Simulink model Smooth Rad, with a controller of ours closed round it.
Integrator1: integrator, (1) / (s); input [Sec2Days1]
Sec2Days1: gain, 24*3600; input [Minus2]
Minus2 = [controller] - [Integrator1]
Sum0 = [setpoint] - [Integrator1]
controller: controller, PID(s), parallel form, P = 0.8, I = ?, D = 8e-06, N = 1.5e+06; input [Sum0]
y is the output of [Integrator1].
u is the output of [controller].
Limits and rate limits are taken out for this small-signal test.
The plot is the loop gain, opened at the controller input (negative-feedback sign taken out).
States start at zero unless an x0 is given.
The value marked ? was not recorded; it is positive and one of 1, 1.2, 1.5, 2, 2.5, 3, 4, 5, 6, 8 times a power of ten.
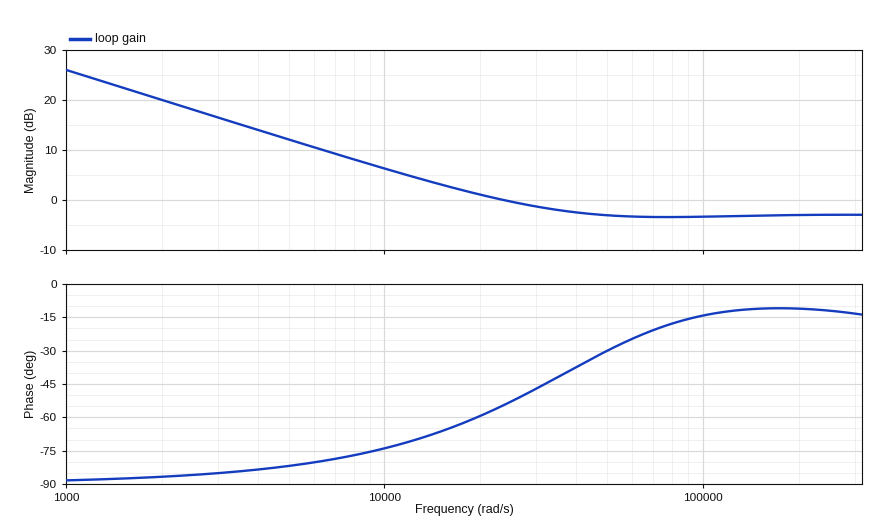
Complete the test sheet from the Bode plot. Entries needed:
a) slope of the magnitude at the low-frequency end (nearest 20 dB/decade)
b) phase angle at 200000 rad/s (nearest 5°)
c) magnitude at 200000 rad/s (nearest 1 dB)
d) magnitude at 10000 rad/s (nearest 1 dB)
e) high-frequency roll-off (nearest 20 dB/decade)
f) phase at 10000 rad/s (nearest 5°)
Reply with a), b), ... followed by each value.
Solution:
a) -20 dB/decade
b) -10°
c) -3 dB
d) 6 dB
e) 0 dB/decade
f) -75°
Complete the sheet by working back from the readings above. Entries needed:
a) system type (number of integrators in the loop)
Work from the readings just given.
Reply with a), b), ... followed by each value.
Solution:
a) 1
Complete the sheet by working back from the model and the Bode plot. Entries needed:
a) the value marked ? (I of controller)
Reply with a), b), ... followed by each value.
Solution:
a) 20000
